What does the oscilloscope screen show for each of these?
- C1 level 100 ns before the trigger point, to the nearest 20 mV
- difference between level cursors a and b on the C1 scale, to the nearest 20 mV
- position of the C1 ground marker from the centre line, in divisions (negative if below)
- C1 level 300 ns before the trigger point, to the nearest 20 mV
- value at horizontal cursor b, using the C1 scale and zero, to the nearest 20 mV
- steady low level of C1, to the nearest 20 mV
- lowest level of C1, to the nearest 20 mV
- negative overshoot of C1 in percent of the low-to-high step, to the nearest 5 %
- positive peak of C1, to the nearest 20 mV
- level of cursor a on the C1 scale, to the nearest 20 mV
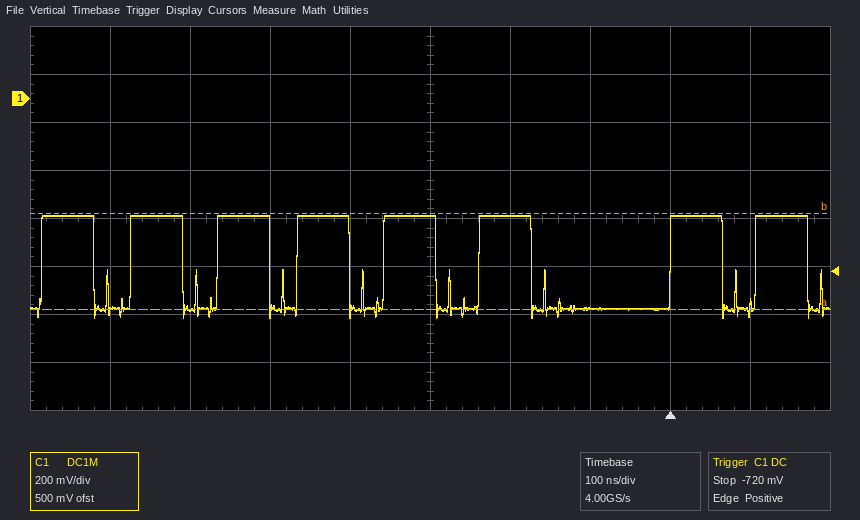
-880 mV
400 mV
+2.5 div
-480 mV
-480 mV
-880 mV
-920 mV
10 %
-480 mV
-880 mV
